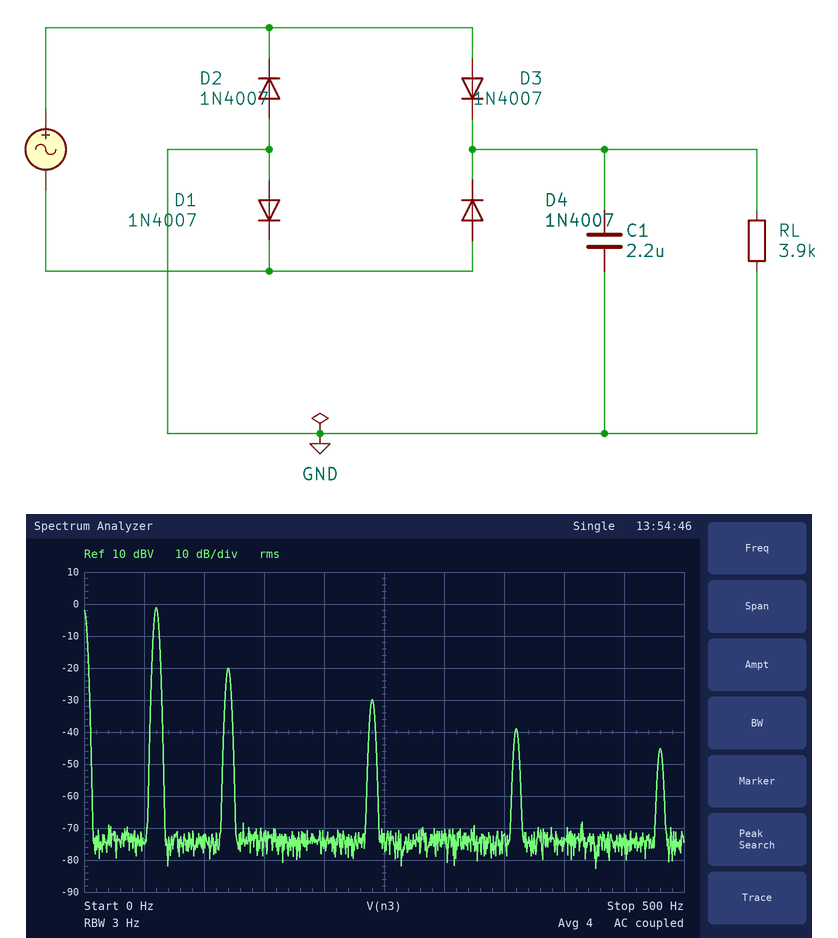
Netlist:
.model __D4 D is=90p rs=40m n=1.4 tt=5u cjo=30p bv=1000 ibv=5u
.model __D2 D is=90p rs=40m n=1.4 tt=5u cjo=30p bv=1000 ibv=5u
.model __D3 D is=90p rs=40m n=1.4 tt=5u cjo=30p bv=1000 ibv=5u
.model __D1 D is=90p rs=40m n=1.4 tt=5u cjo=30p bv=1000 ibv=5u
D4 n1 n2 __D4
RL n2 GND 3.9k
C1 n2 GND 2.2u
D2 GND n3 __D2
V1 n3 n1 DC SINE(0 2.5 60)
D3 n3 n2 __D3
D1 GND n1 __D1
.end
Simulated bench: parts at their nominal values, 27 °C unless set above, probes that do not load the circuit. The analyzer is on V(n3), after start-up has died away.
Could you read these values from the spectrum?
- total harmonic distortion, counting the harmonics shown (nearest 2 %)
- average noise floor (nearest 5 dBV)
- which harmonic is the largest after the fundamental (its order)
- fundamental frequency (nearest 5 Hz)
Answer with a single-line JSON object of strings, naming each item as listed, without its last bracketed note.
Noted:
{"total harmonic distortion, counting the harmonics shown": "12 %", "average noise floor": "-75 dBV", "which harmonic is the largest after the fundamental": "2", "fundamental frequency": "60 Hz"}
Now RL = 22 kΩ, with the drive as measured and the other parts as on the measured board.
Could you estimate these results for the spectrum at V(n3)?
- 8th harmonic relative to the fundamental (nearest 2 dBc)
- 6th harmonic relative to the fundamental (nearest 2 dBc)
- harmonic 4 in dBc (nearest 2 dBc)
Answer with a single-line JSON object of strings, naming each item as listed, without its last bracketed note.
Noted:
{"8th harmonic relative to the fundamental": "-52 dBc", "6th harmonic relative to the fundamental": "-46 dBc", "harmonic 4 in dBc": "-38 dBc"}
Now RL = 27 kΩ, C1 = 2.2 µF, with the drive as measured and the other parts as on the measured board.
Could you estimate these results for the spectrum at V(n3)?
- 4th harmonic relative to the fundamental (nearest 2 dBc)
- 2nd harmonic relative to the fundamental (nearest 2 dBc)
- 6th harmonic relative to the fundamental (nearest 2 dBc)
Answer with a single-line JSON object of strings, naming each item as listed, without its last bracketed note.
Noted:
{"4th harmonic relative to the fundamental": "-40 dBc", "2nd harmonic relative to the fundamental": "-32 dBc", "6th harmonic relative to the fundamental": "-46 dBc"}
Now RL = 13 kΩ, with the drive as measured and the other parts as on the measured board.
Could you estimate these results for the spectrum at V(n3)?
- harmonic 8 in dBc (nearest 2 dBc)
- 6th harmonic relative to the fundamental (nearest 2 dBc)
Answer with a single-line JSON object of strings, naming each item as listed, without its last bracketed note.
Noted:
{"harmonic 8 in dBc": "-48 dBc", "6th harmonic relative to the fundamental": "-42 dBc"}
